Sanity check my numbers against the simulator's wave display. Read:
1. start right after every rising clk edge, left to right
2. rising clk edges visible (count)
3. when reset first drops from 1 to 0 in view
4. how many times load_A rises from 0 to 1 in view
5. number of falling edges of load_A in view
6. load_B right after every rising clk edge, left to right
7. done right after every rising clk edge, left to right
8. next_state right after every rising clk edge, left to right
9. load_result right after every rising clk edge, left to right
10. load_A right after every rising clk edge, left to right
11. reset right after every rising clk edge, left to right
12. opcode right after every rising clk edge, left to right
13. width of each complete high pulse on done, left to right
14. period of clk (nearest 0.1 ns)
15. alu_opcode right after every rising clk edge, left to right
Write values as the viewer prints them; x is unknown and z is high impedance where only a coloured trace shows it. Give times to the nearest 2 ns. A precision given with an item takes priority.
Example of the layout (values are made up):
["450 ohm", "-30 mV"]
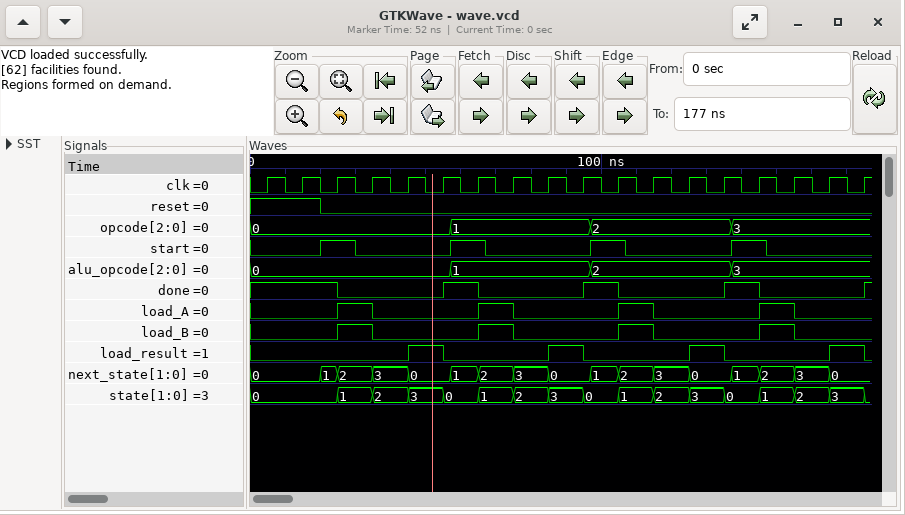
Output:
["0 0 1 0 0 0 1 0 0 0 1 0 0 0 1 0 0 0", "18", "20 ns", "4", "4", "0 0 1 0 0 0 1 0 0 0 1 0 0 0 1 0 0 0", "1 1 0 0 0 1 0 0 0 1 0 0 0 1 0 0 0 1", "0, 0, 2, 3, 0, 0, 2, 3, 0, 0, 2, 3, 0, 0, 2, 3, 0, 0", "0 0 0 0 1 0 0 0 1 0 0 0 1 0 0 0 1 0", "0 0 1 0 0 0 1 0 0 0 1 0 0 0 1 0 0 0", "1 1 0 0 0 0 0 0 0 0 0 0 0 0 0 0 0 0", "0, 0, 0, 0, 0, 0, 1, 1, 1, 1, 2, 2, 2, 2, 3, 3, 3, 3", "10 ns, 10 ns, 10 ns", "10 ns", "0, 0, 0, 0, 0, 0, 1, 1, 1, 1, 2, 2, 2, 2, 3, 3, 3, 3"]
